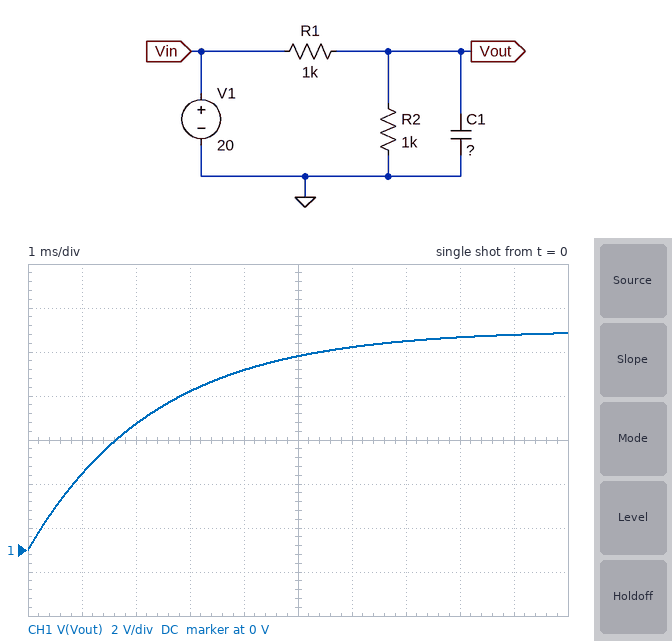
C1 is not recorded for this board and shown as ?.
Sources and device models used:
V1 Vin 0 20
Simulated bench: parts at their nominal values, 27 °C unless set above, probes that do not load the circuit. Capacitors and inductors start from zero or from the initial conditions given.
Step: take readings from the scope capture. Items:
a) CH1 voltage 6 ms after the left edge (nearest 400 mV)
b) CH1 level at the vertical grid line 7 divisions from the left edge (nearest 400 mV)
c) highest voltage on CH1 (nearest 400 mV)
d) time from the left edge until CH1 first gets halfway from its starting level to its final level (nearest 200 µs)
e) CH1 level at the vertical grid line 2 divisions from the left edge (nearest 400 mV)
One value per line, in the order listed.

9.2 V
9.6 V
10.0 V
1.6 ms
5.6 V
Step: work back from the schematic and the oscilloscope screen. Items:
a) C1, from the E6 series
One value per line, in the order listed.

4.7 µF
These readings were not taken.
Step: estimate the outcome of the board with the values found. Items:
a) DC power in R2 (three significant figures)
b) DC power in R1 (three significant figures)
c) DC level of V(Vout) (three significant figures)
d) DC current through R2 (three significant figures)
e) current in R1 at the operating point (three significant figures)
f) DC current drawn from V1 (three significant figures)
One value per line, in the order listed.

100 mW
100 mW
10.0 V
10.0 mA
10.0 mA
10.0 mA
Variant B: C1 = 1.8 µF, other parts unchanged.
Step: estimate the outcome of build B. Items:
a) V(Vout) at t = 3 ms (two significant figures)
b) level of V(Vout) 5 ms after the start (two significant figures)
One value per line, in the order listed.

9.6 V
10 V
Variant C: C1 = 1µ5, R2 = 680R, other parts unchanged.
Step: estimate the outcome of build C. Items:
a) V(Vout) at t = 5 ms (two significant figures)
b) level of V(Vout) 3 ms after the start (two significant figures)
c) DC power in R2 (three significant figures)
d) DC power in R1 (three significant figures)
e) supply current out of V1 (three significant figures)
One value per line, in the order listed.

8.1 V
8.0 V
96.4 mW
142 mW
11.9 mA
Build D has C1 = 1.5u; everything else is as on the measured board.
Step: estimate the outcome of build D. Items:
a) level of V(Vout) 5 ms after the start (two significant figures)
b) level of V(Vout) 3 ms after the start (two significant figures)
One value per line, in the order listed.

10 V
9.8 V
